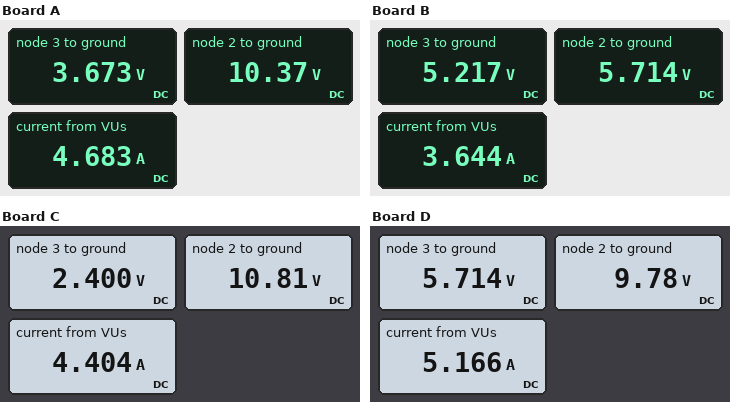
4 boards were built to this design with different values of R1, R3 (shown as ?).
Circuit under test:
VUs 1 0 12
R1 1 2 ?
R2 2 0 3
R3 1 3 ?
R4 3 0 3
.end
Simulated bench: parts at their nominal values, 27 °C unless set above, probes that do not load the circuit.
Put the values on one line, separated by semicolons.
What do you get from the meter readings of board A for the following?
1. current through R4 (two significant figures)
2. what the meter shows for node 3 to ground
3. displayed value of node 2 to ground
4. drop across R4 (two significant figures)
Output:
1.2 A; 3.673 V; 10.37 V; 3.7 V
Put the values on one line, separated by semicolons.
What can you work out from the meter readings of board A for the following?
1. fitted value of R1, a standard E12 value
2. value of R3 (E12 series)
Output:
0.47 Ω; 6.8 Ω
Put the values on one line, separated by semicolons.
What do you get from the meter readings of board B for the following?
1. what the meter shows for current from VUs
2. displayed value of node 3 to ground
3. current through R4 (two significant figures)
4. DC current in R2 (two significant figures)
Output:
3.644 A; 5.217 V; 1.7 A; 1.9 A
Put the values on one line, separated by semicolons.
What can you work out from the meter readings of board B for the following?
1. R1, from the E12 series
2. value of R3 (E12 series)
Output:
3.3 Ω; 3.9 Ω
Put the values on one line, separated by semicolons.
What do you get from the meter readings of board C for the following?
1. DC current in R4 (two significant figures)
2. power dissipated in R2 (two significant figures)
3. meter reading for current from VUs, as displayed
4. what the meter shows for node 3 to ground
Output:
800 mA; 39 W; 4.404 A; 2.400 V
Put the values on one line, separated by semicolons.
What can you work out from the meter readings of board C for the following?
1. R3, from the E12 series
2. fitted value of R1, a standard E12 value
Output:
12 Ω; 0.33 Ω
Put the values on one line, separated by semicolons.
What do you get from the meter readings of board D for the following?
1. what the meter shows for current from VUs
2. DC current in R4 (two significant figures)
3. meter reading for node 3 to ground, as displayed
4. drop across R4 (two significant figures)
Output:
5.166 A; 1.9 A; 5.714 V; 5.7 V
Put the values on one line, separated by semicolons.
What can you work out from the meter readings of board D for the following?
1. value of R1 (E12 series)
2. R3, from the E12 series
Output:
0.68 Ω; 3.3 Ω
